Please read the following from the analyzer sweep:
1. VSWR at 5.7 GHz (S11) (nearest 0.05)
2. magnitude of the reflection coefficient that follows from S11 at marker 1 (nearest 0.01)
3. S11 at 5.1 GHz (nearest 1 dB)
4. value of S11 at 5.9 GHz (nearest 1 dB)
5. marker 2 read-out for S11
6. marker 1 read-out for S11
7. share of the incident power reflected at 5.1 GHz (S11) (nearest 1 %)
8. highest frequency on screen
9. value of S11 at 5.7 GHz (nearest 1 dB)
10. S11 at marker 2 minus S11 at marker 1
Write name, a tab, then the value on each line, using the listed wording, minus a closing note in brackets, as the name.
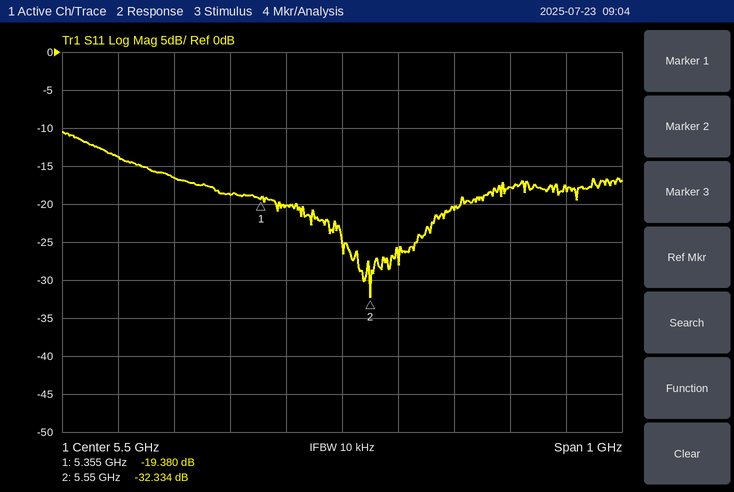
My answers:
VSWR at 5.7 GHz (S11)	1.20
magnitude of the reflection coefficient that follows from S11 at marker 1	0.11
S11 at 5.1 GHz	-14 dB
value of S11 at 5.9 GHz	-18 dB
marker 2 read-out for S11	-32.334 dB
marker 1 read-out for S11	-19.380 dB
share of the incident power reflected at 5.1 GHz (S11)	4 %
highest frequency on screen	6 GHz
value of S11 at 5.7 GHz	-21 dB
S11 at marker 2 minus S11 at marker 1	-12.954 dB
